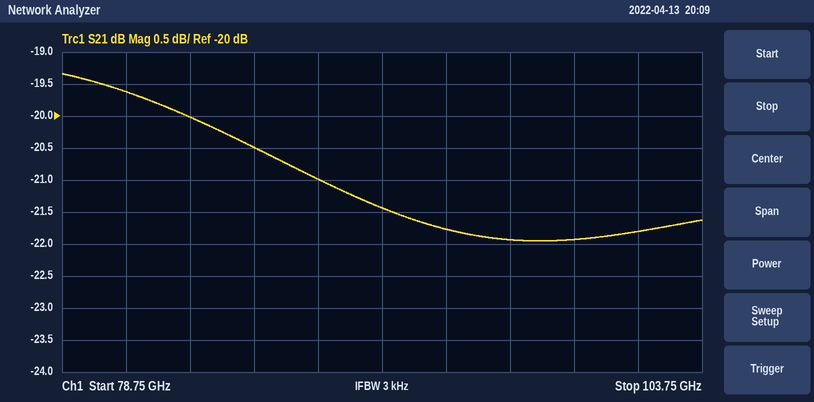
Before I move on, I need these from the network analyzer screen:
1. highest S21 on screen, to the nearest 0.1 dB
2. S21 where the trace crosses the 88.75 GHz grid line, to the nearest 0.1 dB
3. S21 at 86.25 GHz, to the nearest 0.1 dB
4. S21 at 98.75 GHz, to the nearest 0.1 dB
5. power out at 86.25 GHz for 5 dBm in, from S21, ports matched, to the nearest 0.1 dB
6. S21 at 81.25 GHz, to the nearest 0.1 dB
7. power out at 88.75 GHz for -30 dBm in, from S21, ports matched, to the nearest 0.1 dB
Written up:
-19.3 dB
-21.0 dB
-20.5 dB
-21.9 dB
-15.5 dBm
-19.6 dB
-51.0 dBm
